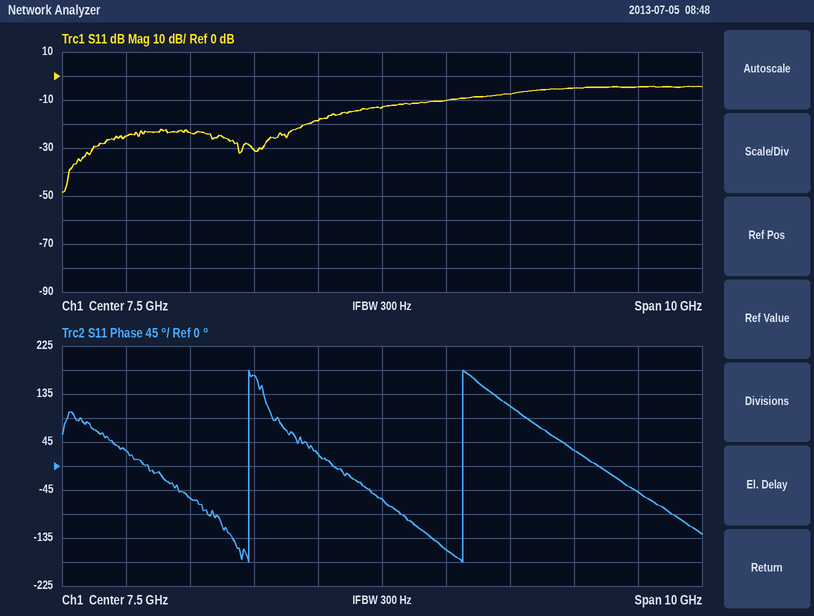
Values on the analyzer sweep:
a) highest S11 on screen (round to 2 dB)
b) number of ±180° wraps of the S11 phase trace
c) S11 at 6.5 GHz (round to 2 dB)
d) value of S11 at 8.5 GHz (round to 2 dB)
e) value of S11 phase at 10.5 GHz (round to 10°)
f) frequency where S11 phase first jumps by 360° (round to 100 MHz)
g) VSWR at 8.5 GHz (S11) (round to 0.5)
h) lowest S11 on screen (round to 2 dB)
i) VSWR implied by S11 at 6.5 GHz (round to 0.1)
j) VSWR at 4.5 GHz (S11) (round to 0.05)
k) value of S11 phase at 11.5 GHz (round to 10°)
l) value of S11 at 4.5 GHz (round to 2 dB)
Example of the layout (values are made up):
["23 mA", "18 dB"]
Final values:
["-4 dB", "2", "-18 dB", "-10 dB", "30°", "5.4 GHz", "2.0", "-48 dB", "1.3", "1.15", "-50°", "-24 dB"]
